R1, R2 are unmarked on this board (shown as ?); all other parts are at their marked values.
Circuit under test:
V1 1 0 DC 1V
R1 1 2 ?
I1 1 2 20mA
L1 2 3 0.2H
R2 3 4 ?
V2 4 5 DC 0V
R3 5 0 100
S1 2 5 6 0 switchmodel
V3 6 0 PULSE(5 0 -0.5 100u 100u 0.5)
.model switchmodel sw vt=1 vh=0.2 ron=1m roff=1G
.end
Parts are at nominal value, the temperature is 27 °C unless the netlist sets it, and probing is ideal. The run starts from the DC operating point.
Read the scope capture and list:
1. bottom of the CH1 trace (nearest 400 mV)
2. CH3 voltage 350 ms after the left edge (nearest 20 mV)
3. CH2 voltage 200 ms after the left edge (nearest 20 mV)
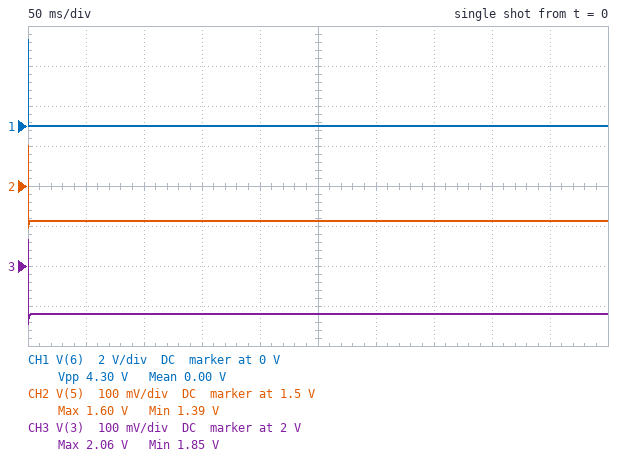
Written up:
0 V
1.88 V
1.42 V
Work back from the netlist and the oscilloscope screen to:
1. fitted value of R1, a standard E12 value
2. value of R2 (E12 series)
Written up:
150 Ω
33 Ω
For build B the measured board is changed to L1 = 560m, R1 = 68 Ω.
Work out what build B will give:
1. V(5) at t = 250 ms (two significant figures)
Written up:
1.2 V
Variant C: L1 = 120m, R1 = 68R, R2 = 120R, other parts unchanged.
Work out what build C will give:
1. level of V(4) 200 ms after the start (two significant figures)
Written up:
820 mV
